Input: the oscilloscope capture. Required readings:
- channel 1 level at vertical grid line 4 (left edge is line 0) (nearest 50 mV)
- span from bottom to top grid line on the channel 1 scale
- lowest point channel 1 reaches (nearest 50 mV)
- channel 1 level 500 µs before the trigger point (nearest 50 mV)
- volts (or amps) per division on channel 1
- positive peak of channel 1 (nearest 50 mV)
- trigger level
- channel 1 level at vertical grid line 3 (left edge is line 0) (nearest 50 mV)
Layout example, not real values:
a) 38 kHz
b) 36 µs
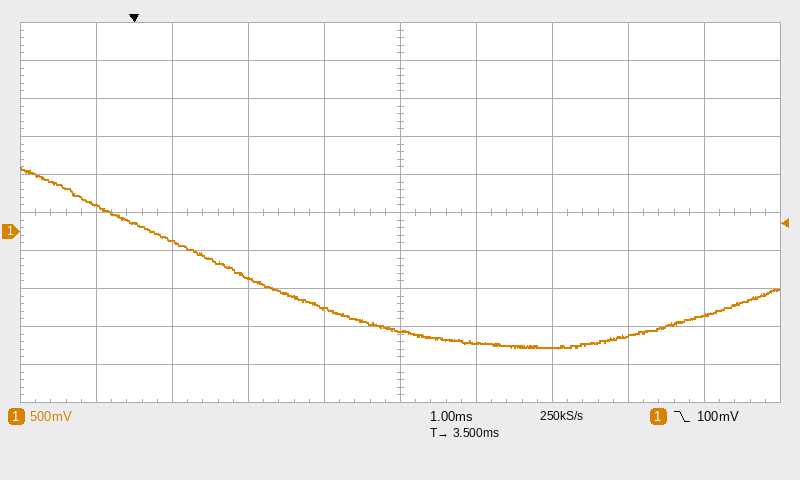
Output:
a) -1.00 V
b) 5 V
c) -1.55 V
d) 350 mV
e) 500 mV
f) 850 mV
g) 100 mV
h) -600 mV
